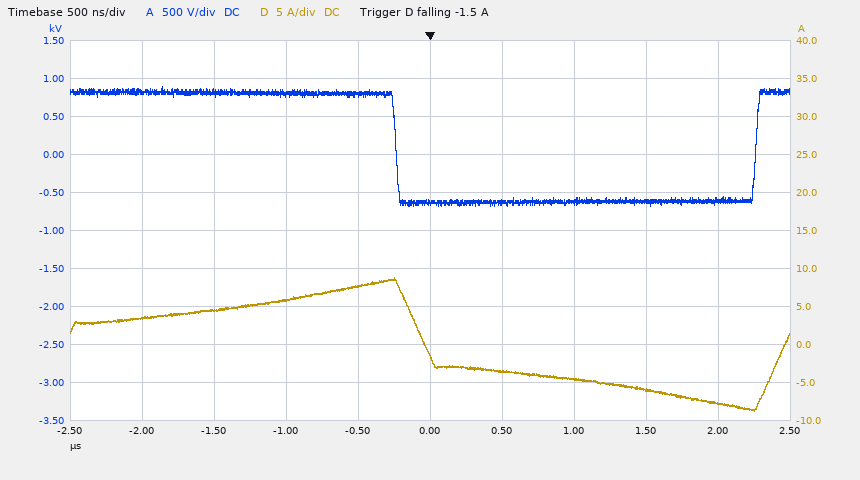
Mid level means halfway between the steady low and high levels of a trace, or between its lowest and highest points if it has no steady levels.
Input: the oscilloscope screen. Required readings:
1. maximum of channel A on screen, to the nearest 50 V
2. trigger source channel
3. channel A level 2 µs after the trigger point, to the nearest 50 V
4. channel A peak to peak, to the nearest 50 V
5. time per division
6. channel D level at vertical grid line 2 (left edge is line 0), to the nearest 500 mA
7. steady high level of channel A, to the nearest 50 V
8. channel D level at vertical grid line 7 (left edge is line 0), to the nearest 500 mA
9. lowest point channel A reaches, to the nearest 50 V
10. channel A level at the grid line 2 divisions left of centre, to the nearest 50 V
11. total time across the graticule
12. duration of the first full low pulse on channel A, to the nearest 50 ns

900 V
channel D
-600 V
1.60 kV
500 ns
4.5 A
800 V
-4.5 A
-700 V
800 V
5 µs
2.50 µs
